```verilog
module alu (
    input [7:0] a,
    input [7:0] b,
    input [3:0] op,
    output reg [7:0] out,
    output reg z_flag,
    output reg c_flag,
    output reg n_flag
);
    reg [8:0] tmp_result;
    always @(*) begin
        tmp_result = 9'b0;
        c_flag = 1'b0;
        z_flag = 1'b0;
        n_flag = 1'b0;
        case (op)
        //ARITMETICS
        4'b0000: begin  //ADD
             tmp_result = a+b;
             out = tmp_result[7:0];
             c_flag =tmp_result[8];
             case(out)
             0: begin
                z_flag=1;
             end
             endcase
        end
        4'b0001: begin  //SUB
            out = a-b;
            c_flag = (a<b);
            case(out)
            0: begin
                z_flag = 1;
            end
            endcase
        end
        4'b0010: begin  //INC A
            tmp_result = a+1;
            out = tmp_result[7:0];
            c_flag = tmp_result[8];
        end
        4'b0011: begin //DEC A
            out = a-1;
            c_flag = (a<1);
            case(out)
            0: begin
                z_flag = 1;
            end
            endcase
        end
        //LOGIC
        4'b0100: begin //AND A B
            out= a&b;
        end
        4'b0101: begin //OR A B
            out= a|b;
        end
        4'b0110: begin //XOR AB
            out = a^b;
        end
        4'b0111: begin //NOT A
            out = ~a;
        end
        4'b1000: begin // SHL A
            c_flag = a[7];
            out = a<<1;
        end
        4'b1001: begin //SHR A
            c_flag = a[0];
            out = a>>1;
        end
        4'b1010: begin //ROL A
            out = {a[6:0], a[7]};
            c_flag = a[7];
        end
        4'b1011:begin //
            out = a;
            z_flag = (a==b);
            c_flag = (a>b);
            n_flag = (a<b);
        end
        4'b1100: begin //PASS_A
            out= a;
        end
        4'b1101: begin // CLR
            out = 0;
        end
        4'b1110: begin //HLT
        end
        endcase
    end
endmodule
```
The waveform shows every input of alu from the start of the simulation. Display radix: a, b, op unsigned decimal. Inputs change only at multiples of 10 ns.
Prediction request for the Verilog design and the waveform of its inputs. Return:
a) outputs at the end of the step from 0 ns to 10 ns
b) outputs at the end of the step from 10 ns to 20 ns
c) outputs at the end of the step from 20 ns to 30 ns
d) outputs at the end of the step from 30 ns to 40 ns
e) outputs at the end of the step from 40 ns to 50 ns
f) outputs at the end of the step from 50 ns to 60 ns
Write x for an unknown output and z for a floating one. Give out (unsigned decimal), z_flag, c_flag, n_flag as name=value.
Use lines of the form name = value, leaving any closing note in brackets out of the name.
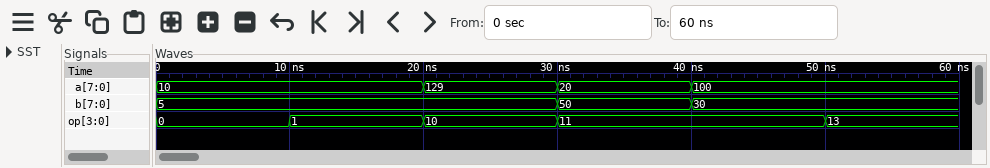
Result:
outputs at the end of the step from 0 ns to 10 ns = out=15, z_flag=0, c_flag=0, n_flag=0
outputs at the end of the step from 10 ns to 20 ns = out=5, z_flag=0, c_flag=0, n_flag=0
outputs at the end of the step from 20 ns to 30 ns = out=3, z_flag=0, c_flag=1, n_flag=0
outputs at the end of the step from 30 ns to 40 ns = out=20, z_flag=0, c_flag=0, n_flag=1
outputs at the end of the step from 40 ns to 50 ns = out=100, z_flag=0, c_flag=1, n_flag=0
outputs at the end of the step from 50 ns to 60 ns = out=0, z_flag=0, c_flag=0, n_flag=0
